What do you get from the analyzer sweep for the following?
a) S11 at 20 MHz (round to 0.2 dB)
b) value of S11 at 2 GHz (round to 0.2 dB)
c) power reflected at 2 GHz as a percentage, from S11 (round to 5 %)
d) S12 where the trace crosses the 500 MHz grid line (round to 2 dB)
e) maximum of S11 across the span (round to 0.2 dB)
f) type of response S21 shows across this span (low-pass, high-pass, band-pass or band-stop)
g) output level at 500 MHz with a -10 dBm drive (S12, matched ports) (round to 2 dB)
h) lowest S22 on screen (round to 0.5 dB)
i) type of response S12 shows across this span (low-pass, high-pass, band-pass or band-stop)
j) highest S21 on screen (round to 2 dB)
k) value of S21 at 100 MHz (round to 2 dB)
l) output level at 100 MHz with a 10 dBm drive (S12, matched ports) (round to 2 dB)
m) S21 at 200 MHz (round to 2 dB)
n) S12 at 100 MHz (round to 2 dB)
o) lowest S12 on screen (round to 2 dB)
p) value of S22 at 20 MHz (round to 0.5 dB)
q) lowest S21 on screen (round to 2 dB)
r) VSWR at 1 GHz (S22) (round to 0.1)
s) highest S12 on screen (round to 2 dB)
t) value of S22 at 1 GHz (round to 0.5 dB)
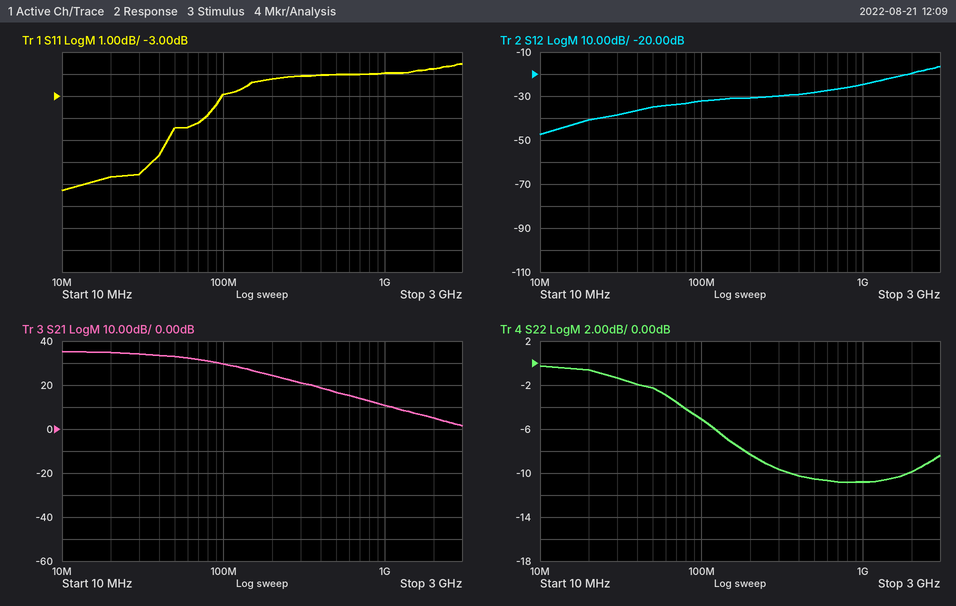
-6.6 dB
-1.8 dB
65 %
-28 dB
-1.6 dB
low-pass
-38 dBm
-11.0 dB
high-pass
36 dB
30 dB
-22 dBm
24 dB
-32 dB
-48 dB
-0.5 dB
2 dB
1.8
-16 dB
-11.0 dB
